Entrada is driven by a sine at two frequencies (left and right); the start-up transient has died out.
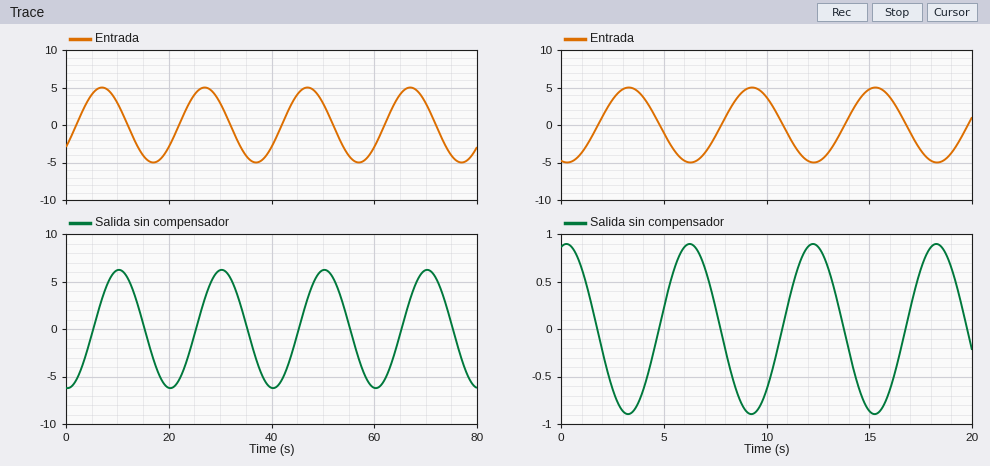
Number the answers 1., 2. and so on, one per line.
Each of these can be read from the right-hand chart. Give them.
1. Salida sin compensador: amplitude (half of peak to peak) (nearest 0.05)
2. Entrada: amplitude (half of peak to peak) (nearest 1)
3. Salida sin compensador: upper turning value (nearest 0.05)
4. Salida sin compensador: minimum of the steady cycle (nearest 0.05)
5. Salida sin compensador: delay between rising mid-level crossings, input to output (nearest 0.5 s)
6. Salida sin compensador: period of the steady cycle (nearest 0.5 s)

1. 0.90
2. 5
3. 0.90
4. -0.90
5. 3.0 s
6. 6.0 s
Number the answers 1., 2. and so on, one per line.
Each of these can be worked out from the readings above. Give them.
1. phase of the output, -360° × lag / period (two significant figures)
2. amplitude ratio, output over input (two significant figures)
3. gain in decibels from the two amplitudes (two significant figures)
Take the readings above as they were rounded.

1. -180°
2. 0.18
3. -15 dB
